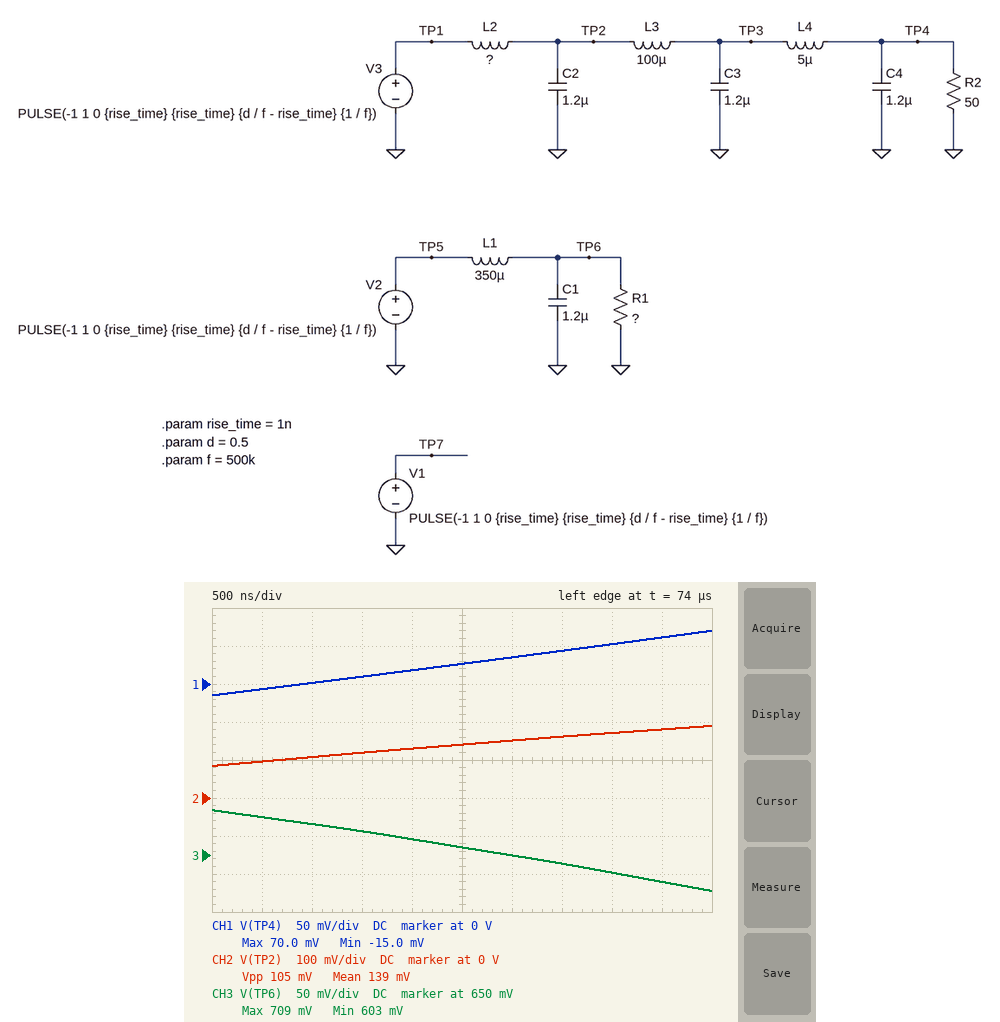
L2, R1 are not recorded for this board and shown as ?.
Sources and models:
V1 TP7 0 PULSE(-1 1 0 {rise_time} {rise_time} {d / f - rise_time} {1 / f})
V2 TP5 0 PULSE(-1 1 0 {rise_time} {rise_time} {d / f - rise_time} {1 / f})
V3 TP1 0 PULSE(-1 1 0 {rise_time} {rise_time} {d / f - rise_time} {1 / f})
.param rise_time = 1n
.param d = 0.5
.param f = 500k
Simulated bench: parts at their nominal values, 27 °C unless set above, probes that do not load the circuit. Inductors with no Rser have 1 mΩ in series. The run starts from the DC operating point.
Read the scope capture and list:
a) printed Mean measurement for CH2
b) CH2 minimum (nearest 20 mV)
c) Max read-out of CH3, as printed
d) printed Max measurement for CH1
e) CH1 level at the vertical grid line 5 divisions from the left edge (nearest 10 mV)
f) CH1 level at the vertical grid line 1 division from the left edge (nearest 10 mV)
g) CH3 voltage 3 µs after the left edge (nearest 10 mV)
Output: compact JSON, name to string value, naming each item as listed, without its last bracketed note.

{"printed Mean measurement for CH2": "139 mV", "CH2 minimum": "80 mV", "Max read-out of CH3, as printed": "709 mV", "printed Max measurement for CH1": "70.0 mV", "CH1 level at the vertical grid line 5 divisions from the left edge": "30 mV", "CH1 level at the vertical grid line 1 division from the left edge": "-10 mV", "CH3 voltage 3 µs after the left edge": "650 mV"}
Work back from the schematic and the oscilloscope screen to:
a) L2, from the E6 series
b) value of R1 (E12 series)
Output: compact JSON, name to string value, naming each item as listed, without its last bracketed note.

{"L2, from the E6 series": "470 µH", "value of R1": "120 Ω"}
